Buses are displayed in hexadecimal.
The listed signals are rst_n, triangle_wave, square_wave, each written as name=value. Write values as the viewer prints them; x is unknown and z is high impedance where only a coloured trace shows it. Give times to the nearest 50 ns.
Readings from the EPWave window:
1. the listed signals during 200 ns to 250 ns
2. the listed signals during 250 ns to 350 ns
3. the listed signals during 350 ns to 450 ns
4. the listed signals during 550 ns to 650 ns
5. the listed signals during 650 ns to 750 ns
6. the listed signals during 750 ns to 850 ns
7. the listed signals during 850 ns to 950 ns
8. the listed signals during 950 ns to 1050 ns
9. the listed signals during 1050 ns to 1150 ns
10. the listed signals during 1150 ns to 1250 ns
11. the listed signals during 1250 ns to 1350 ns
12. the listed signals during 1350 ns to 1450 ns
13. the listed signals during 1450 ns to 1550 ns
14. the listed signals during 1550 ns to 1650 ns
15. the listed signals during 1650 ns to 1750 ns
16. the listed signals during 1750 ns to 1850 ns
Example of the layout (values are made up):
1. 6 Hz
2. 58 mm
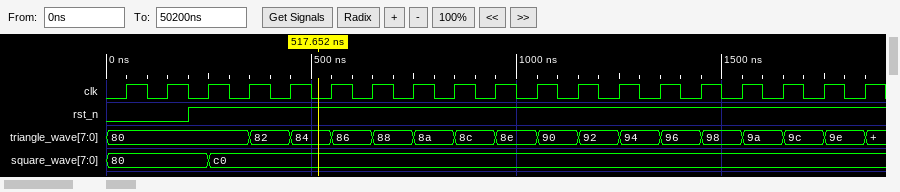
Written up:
1. rst_n=1, triangle_wave=80, square_wave=80
2. rst_n=1, triangle_wave=80, square_wave=c0
3. rst_n=1, triangle_wave=82, square_wave=c0
4. rst_n=1, triangle_wave=86, square_wave=c0
5. rst_n=1, triangle_wave=88, square_wave=c0
6. rst_n=1, triangle_wave=8a, square_wave=c0
7. rst_n=1, triangle_wave=8c, square_wave=c0
8. rst_n=1, triangle_wave=8e, square_wave=c0
9. rst_n=1, triangle_wave=90, square_wave=c0
10. rst_n=1, triangle_wave=92, square_wave=c0
11. rst_n=1, triangle_wave=94, square_wave=c0
12. rst_n=1, triangle_wave=96, square_wave=c0
13. rst_n=1, triangle_wave=98, square_wave=c0
14. rst_n=1, triangle_wave=9a, square_wave=c0
15. rst_n=1, triangle_wave=9c, square_wave=c0
16. rst_n=1, triangle_wave=9e, square_wave=c0
